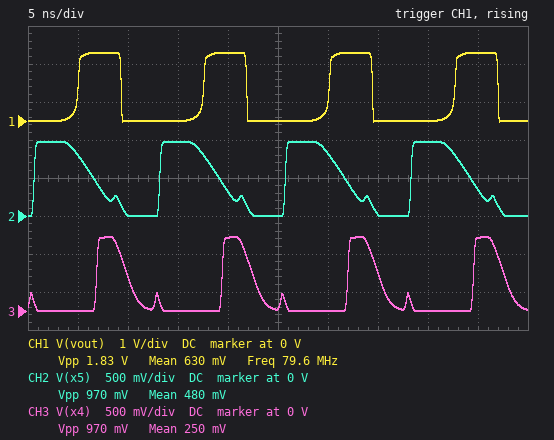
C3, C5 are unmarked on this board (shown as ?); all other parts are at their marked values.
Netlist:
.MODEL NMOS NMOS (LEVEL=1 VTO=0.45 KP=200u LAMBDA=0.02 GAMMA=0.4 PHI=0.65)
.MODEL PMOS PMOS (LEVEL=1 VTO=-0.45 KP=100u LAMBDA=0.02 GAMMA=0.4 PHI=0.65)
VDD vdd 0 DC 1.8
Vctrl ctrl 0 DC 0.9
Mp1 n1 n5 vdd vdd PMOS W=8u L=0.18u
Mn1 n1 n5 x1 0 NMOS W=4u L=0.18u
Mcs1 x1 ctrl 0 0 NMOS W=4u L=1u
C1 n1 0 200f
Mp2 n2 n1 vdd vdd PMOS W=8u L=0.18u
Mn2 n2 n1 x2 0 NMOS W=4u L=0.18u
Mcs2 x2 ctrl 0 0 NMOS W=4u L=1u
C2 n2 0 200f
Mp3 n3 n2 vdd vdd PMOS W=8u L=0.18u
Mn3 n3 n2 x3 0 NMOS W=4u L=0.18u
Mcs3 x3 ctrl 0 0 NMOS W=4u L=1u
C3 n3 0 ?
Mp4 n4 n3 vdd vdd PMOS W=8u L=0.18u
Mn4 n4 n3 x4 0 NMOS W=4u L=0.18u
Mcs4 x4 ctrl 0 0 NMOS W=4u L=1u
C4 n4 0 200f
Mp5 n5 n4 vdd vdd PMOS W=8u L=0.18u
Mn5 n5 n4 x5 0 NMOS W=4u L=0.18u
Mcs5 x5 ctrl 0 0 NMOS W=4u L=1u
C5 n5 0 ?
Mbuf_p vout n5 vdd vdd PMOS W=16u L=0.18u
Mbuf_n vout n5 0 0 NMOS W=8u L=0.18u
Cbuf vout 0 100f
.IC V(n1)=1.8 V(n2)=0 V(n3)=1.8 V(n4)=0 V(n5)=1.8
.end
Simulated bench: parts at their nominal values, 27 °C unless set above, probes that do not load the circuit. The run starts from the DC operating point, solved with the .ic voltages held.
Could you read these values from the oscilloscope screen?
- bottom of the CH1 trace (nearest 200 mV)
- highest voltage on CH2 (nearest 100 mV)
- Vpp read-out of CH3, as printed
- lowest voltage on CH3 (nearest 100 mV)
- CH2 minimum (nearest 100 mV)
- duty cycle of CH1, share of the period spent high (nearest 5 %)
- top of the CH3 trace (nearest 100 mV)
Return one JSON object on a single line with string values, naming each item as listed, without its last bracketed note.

{"bottom of the CH1 trace": "0 V", "highest voltage on CH2": "1.0 V", "Vpp read-out of CH3, as printed": "970 mV", "lowest voltage on CH3": "0 V", "CH2 minimum": "0 V", "duty cycle of CH1, share of the period spent high": "35 %", "top of the CH3 trace": "1.0 V"}
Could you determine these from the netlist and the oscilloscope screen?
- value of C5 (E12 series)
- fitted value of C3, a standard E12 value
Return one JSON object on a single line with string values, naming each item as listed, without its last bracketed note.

{"value of C5": "390 fF", "fitted value of C3, a standard E12 value": "120 fF"}
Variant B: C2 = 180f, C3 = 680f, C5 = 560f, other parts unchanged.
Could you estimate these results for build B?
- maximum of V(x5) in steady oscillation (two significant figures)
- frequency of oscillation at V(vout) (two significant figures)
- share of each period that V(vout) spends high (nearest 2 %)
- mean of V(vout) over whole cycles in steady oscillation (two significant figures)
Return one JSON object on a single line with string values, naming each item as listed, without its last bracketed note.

{"maximum of V(x5) in steady oscillation": "970 mV", "frequency of oscillation at V(vout)": "51 MHz", "share of each period that V(vout) spends high": "22 %", "mean of V(vout) over whole cycles in steady oscillation": "410 mV"}
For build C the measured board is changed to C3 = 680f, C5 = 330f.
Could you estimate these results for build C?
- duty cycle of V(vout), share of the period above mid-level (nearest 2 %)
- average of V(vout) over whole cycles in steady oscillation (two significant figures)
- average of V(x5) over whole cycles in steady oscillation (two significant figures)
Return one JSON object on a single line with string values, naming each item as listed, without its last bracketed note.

{"duty cycle of V(vout), share of the period above mid-level": "28 %", "average of V(vout) over whole cycles in steady oscillation": "510 mV", "average of V(x5) over whole cycles in steady oscillation": "290 mV"}
